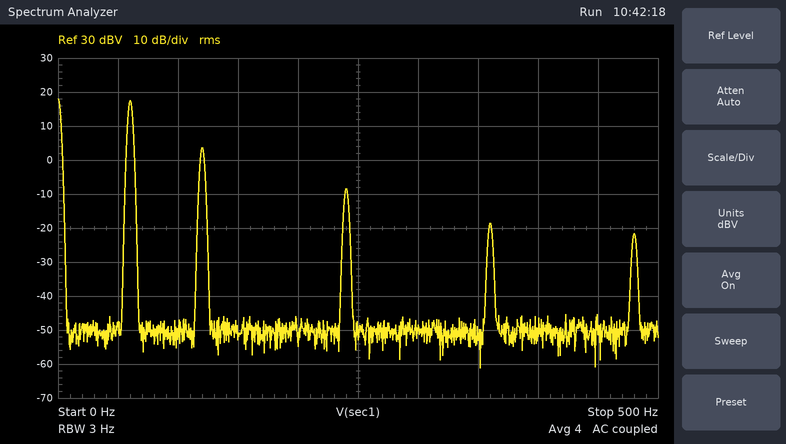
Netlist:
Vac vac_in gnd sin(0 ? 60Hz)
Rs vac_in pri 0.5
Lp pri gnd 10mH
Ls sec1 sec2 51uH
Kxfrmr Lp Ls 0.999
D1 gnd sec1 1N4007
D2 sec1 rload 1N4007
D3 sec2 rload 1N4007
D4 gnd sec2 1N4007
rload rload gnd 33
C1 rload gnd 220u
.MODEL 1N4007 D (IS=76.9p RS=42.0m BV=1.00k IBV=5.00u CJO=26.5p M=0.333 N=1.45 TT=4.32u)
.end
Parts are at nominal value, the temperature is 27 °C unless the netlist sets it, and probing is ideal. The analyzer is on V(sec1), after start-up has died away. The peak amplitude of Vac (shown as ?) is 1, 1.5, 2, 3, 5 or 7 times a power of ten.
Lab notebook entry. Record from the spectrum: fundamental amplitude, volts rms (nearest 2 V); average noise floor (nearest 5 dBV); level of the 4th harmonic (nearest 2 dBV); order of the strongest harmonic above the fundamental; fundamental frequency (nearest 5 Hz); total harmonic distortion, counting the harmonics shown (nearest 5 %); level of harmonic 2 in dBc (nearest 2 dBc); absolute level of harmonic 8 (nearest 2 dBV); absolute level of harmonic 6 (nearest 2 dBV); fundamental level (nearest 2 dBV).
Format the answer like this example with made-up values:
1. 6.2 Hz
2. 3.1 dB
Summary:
1. 8 V
2. -50 dBV
3. -8 dBV
4. 2
5. 60 Hz
6. 20 %
7. -14 dBc
8. -22 dBV
9. -18 dBV
10. 18 dBV
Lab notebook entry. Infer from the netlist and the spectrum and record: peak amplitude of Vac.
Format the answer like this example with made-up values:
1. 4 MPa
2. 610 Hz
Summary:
1. 300 V
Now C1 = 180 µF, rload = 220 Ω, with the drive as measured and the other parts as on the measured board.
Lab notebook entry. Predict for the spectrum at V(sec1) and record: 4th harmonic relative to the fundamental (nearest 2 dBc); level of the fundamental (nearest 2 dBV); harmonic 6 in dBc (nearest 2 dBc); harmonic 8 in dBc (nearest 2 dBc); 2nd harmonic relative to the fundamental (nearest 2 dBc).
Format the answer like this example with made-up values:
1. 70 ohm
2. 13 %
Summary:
1. -32 dBc
2. 18 dBV
3. -38 dBc
4. -44 dBc
5. -26 dBc
